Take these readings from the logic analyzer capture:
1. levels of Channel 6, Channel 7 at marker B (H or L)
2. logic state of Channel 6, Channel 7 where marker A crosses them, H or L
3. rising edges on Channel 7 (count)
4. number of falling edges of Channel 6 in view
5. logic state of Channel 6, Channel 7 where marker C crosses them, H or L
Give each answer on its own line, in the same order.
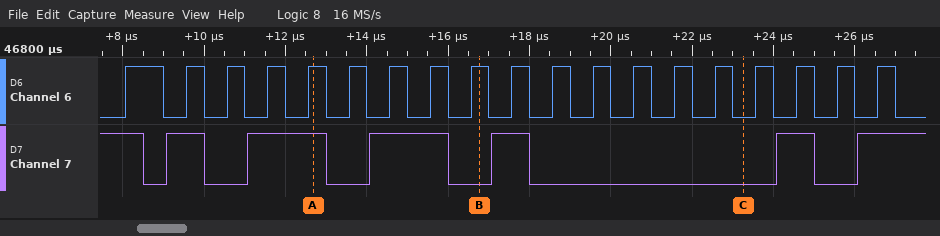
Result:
Channel 6=H, Channel 7=L
Channel 6=H, Channel 7=H
6
19
Channel 6=L, Channel 7=L
